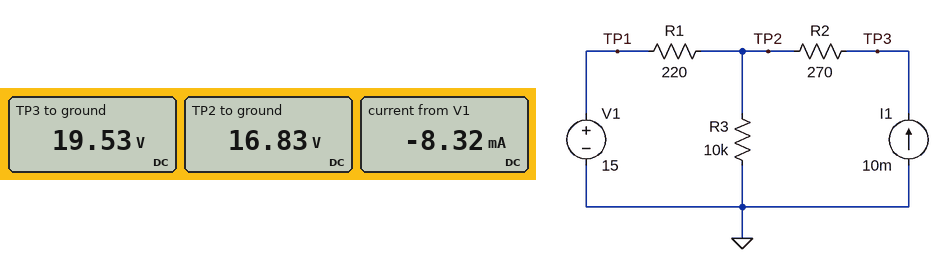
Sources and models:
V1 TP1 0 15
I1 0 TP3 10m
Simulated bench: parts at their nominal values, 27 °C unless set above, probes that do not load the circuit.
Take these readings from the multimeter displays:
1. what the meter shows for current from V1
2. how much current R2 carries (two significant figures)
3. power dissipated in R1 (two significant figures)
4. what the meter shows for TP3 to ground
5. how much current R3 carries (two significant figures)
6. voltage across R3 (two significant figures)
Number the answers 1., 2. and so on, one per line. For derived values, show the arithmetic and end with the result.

1. -8.32 mA
2. (19.53 V - 16.83 V) / 270 Ω = 10 mA
3. (16.83 V - 15 V)^2 / 220 Ω = 15 mW
4. 19.53 V
5. (16.83 V) / 10 kΩ = 1.7 mA
6. 16.83 V = 17 V
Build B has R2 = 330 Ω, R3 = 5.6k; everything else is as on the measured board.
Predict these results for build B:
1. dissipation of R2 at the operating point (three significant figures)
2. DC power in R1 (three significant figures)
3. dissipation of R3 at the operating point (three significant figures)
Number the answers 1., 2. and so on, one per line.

1. 33.0 mW
2. 10.9 mW
3. 48.9 mW
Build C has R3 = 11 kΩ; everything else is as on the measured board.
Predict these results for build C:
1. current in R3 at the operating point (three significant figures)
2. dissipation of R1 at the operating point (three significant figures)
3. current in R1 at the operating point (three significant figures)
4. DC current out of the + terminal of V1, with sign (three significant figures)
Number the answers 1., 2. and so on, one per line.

1. 1.53 mA
2. 15.8 mW
3. 8.47 mA
4. -8.47 mA
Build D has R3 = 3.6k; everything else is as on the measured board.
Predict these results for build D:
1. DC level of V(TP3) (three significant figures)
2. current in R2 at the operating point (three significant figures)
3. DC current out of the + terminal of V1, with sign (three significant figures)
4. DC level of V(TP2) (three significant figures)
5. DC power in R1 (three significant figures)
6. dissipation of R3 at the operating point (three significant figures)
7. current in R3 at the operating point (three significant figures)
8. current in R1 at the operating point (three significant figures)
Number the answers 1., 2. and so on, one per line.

1. 18.9 V
2. 10.0 mA
3. -5.50 mA
4. 16.2 V
5. 6.65 mW
6. 73.0 mW
7. 4.50 mA
8. 5.50 mA
